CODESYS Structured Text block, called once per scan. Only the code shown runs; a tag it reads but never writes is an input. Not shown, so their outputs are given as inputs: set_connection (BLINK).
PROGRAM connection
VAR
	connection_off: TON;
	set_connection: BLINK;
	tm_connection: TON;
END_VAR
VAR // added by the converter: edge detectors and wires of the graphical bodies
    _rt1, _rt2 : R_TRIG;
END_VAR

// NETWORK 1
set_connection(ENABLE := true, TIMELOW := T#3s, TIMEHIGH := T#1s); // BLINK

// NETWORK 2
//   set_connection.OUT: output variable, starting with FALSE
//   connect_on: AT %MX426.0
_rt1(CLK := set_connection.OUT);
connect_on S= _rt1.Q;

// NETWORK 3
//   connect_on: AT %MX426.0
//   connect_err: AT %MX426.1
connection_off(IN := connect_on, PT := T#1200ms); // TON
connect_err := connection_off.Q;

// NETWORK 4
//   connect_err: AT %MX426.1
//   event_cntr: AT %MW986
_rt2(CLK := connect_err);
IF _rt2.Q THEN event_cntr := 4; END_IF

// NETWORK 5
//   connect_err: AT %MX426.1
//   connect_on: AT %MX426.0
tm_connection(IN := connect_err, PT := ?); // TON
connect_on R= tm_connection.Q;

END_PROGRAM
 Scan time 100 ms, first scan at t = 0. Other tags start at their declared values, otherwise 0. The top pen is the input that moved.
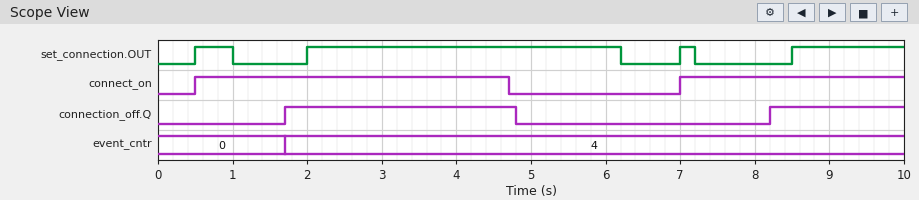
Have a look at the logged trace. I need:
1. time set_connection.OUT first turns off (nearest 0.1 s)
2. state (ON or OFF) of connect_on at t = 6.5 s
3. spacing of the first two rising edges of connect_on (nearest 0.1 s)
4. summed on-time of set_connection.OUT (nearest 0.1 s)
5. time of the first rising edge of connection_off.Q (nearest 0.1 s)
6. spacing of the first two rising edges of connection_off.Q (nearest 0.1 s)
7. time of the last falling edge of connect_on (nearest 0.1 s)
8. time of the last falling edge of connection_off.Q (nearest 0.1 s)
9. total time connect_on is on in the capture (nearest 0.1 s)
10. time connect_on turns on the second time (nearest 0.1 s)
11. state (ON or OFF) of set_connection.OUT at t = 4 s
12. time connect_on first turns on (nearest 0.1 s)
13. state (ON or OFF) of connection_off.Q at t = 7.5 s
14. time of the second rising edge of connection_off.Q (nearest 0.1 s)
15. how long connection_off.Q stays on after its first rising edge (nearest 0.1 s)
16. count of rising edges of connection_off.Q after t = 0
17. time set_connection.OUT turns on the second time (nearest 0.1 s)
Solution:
1.0 s
OFF
6.5 s
6.4 s
1.7 s
6.5 s
4.7 s
4.8 s
7.2 s
7.0 s
ON
0.5 s
OFF
8.2 s
3.1 s
2
2.0 s
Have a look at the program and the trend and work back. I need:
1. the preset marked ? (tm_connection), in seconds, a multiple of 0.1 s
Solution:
3.0 s
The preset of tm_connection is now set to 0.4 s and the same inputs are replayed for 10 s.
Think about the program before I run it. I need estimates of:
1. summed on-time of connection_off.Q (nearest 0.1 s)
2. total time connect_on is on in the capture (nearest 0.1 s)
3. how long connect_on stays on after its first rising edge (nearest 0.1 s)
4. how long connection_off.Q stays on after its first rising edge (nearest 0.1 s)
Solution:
1.0 s
3.2 s
1.6 s
0.5 s
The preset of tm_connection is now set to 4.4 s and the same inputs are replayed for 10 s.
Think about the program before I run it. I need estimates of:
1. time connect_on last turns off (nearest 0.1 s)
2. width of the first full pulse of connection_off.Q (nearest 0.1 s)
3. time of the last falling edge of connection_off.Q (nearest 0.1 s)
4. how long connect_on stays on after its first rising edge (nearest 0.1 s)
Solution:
6.1 s
4.5 s
6.2 s
5.6 s
